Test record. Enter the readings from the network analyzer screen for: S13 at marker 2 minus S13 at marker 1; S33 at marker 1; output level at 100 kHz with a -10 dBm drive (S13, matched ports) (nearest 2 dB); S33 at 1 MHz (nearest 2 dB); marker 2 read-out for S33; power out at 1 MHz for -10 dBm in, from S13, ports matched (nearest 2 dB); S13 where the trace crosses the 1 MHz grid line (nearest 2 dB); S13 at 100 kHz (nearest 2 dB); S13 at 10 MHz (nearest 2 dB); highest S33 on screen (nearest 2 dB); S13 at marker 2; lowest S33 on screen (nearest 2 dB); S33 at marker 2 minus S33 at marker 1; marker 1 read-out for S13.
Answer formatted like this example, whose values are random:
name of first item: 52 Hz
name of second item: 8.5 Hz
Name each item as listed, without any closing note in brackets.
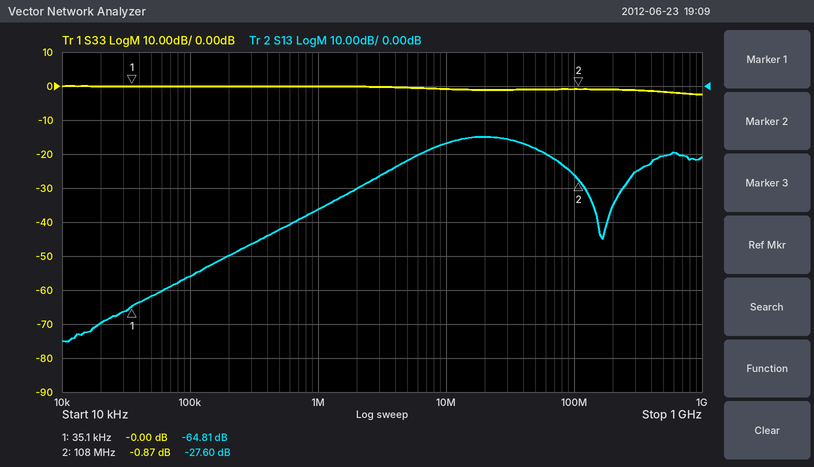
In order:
S13 at marker 2 minus S13 at marker 1: 37.21 dB
S33 at marker 1: -0.00 dB
output level at 100 kHz with a -10 dBm drive (S13, matched ports): -66 dBm
S33 at 1 MHz: 0 dB
marker 2 read-out for S33: -0.87 dB
power out at 1 MHz for -10 dBm in, from S13, ports matched: -46 dBm
S13 where the trace crosses the 1 MHz grid line: -36 dB
S13 at 100 kHz: -56 dB
S13 at 10 MHz: -16 dB
highest S33 on screen: 0 dB
S13 at marker 2: -27.60 dB
lowest S33 on screen: -2 dB
S33 at marker 2 minus S33 at marker 1: -0.87 dB
marker 1 read-out for S13: -64.81 dB
